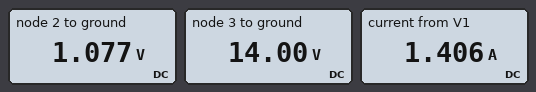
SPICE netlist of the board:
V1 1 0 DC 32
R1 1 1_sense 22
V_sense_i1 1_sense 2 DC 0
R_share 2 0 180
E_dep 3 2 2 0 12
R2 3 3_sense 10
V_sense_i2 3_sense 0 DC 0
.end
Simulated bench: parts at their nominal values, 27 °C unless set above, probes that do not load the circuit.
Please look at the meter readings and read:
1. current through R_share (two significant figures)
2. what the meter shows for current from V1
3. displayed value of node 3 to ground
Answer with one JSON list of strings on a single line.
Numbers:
["6.0 mA", "1.406 A", "14.00 V"]
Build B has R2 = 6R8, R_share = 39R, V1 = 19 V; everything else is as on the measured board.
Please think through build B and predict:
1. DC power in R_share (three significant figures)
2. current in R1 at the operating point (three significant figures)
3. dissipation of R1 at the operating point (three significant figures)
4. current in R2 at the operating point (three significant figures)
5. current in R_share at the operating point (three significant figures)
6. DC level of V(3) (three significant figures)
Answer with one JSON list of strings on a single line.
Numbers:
["4.86 mW", "844 mA", "15.7 W", "833 mA", "11.2 mA", "5.66 V"]
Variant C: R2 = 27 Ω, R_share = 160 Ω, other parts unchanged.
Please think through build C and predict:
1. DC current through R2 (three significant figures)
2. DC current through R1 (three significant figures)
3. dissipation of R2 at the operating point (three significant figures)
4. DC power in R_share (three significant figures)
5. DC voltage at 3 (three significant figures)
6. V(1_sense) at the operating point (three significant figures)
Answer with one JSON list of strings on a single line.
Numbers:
["1.31 A", "1.33 A", "46.6 W", "46.5 mW", "35.5 V", "2.73 V"]
